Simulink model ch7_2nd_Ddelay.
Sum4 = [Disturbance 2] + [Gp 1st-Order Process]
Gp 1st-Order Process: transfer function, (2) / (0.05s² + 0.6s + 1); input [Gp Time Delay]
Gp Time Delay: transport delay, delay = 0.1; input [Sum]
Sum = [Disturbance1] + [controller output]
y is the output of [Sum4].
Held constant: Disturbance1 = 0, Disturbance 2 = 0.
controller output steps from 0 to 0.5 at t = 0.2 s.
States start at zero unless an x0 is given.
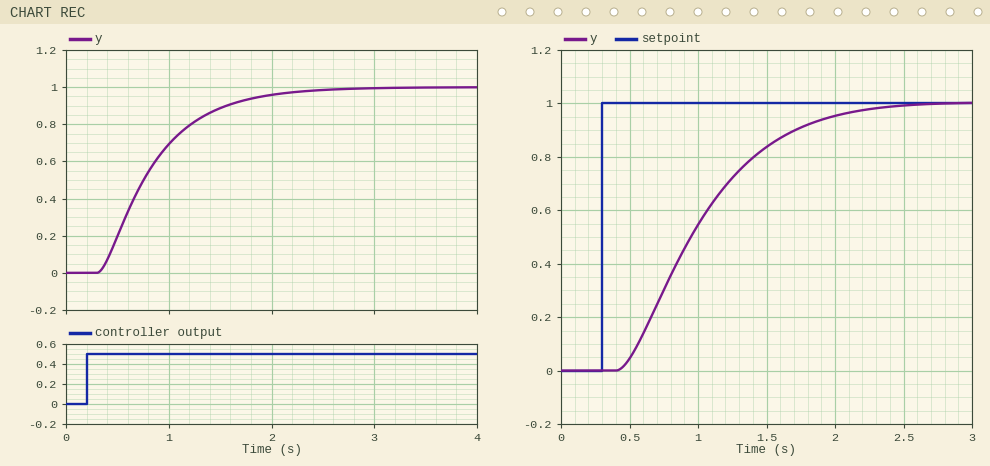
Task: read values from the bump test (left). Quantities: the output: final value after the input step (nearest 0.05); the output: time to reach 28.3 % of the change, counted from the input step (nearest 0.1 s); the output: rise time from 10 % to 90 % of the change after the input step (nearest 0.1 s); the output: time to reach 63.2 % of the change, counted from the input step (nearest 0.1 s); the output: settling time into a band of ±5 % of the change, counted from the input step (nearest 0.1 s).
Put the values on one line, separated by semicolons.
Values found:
1.00; 0.4 s; 1.1 s; 0.7 s; 1.7 s
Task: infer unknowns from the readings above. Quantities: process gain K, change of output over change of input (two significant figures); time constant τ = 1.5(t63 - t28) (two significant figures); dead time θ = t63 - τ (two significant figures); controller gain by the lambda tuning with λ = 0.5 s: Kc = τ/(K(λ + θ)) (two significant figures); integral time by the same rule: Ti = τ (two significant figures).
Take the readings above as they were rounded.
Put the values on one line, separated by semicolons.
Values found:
2.0; 0.45 s; 0.25 s; 0.30; 0.45 s
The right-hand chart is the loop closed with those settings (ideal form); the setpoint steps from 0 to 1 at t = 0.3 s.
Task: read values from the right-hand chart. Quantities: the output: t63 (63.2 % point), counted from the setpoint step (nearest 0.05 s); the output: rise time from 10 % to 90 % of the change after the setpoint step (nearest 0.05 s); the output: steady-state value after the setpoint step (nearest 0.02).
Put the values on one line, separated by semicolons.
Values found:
0.80 s; 1.15 s; 1.00
